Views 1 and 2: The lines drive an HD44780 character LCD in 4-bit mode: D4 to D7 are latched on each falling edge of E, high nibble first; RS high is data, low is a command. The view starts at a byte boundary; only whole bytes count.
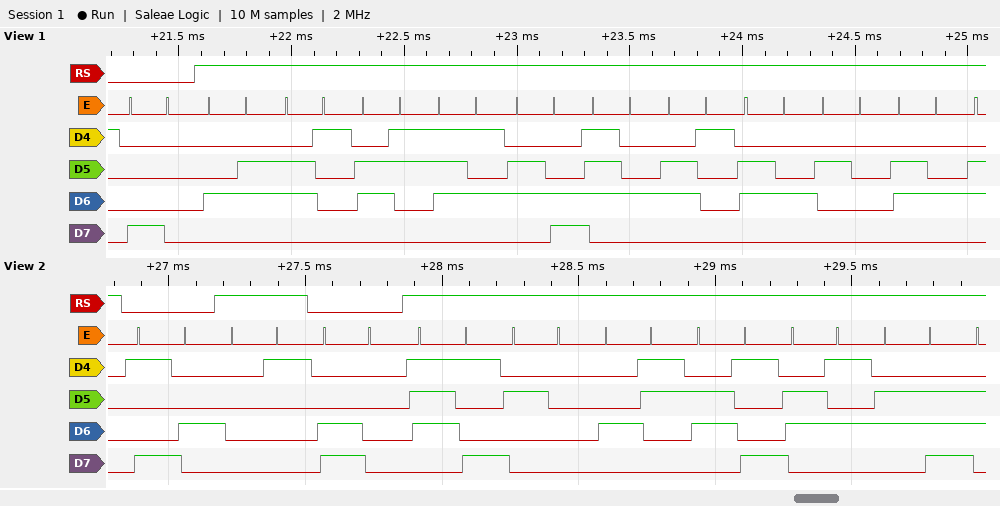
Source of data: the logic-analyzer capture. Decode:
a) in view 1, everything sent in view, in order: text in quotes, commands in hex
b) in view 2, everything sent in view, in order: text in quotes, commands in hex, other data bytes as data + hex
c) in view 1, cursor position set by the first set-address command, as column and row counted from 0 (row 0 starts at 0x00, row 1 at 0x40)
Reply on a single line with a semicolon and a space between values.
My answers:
0x80 "Facultad d"; 0x94 data 01 0xC0 "y Cien"; column 0, row 0
